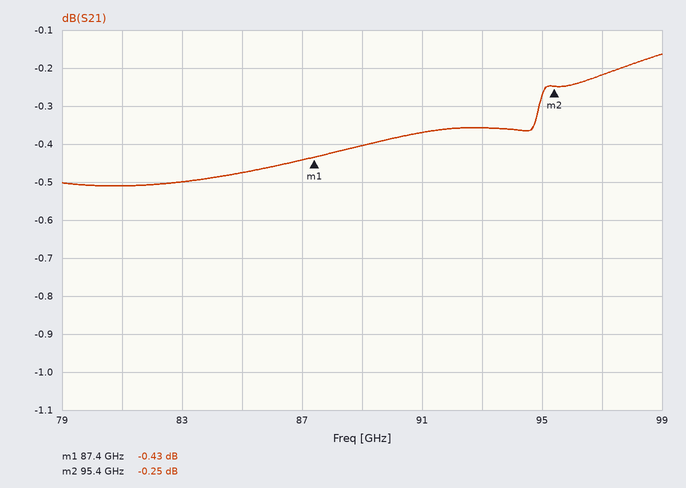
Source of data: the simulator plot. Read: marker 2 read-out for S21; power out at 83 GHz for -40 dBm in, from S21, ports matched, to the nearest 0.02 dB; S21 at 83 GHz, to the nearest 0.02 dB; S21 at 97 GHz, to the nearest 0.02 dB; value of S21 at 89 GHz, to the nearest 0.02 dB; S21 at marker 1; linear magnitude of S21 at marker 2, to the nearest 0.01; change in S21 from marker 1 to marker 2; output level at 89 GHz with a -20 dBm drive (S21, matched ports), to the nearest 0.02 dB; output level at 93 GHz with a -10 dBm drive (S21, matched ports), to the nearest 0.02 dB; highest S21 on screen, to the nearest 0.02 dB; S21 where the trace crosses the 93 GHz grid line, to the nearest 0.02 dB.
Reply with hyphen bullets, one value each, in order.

- -0.25 dB
- -40.50 dBm
- -0.50 dB
- -0.22 dB
- -0.40 dB
- -0.43 dB
- 0.97
- 0.18 dB
- -20.40 dBm
- -10.36 dBm
- -0.16 dB
- -0.36 dB
